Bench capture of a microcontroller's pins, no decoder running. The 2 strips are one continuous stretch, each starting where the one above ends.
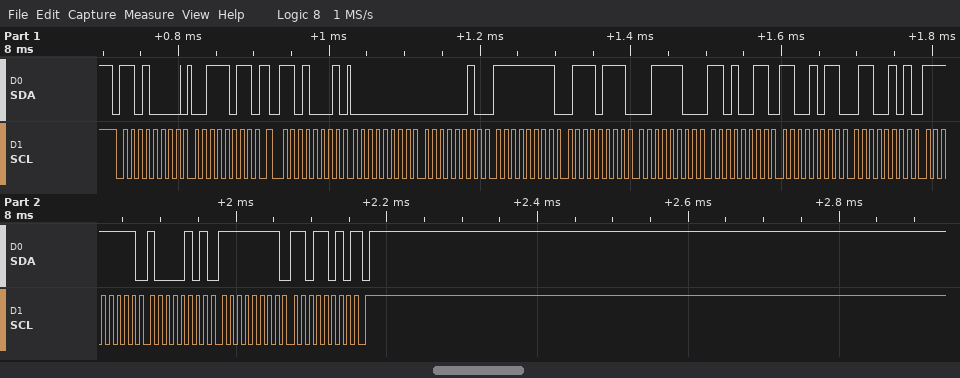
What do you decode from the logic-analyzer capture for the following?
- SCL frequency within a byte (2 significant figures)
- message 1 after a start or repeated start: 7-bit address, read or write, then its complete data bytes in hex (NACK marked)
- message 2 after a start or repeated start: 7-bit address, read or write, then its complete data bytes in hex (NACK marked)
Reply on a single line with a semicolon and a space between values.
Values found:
100 kHz; 0x68 write: 3B; 0x68 read: 00 02 FF 77 3C D3 CB 65 FF 85 FF DA NACK
